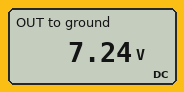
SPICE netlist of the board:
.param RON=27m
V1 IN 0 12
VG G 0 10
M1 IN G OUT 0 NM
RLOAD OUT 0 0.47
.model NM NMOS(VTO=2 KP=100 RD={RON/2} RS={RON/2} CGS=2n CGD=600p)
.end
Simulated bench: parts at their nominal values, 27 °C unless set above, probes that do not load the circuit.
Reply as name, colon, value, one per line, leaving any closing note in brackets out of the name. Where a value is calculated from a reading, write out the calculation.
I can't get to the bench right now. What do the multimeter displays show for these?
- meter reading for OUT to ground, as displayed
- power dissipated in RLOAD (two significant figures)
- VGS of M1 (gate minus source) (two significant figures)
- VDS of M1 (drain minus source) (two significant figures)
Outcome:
meter reading for OUT to ground, as displayed: 7.24 V
power dissipated in RLOAD: (7.24 V)^2 / 470 mΩ = 110 W
VGS of M1 (gate minus source): 10 V - 7.24 V = 2.8 V
VDS of M1 (drain minus source): 12 V - 7.24 V = 4.8 V
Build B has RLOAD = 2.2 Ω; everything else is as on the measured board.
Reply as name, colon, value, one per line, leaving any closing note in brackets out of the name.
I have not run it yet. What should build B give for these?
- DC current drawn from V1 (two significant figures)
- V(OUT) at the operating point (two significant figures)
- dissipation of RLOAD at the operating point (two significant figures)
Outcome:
DC current drawn from V1: 3.5 A
V(OUT) at the operating point: 7.7 V
dissipation of RLOAD at the operating point: 27 W
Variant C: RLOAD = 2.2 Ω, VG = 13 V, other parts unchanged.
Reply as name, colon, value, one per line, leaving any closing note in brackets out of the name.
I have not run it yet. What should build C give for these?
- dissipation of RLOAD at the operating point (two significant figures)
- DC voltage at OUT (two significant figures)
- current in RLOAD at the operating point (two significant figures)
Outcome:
dissipation of RLOAD at the operating point: 51 W
DC voltage at OUT: 11 V
current in RLOAD at the operating point: 4.8 A
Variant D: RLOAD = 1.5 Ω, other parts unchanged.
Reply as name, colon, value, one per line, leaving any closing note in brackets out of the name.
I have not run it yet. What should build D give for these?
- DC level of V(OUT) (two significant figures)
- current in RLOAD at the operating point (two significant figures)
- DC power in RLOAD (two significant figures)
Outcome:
DC level of V(OUT): 7.6 V
current in RLOAD at the operating point: 5.1 A
DC power in RLOAD: 39 W
